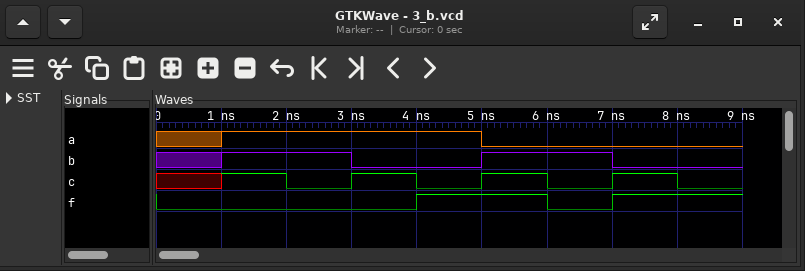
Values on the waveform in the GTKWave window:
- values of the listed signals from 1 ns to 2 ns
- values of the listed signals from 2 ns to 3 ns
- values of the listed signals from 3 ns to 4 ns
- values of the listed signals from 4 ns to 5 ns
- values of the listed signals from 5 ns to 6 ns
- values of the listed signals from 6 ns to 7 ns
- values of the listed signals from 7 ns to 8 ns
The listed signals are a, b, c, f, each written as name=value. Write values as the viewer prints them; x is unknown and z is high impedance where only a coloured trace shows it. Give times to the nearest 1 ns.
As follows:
a=1, b=1, c=1, f=0
a=1, b=1, c=0, f=0
a=1, b=0, c=1, f=0
a=1, b=0, c=0, f=1
a=0, b=1, c=1, f=1
a=0, b=1, c=0, f=0
a=0, b=0, c=1, f=1
